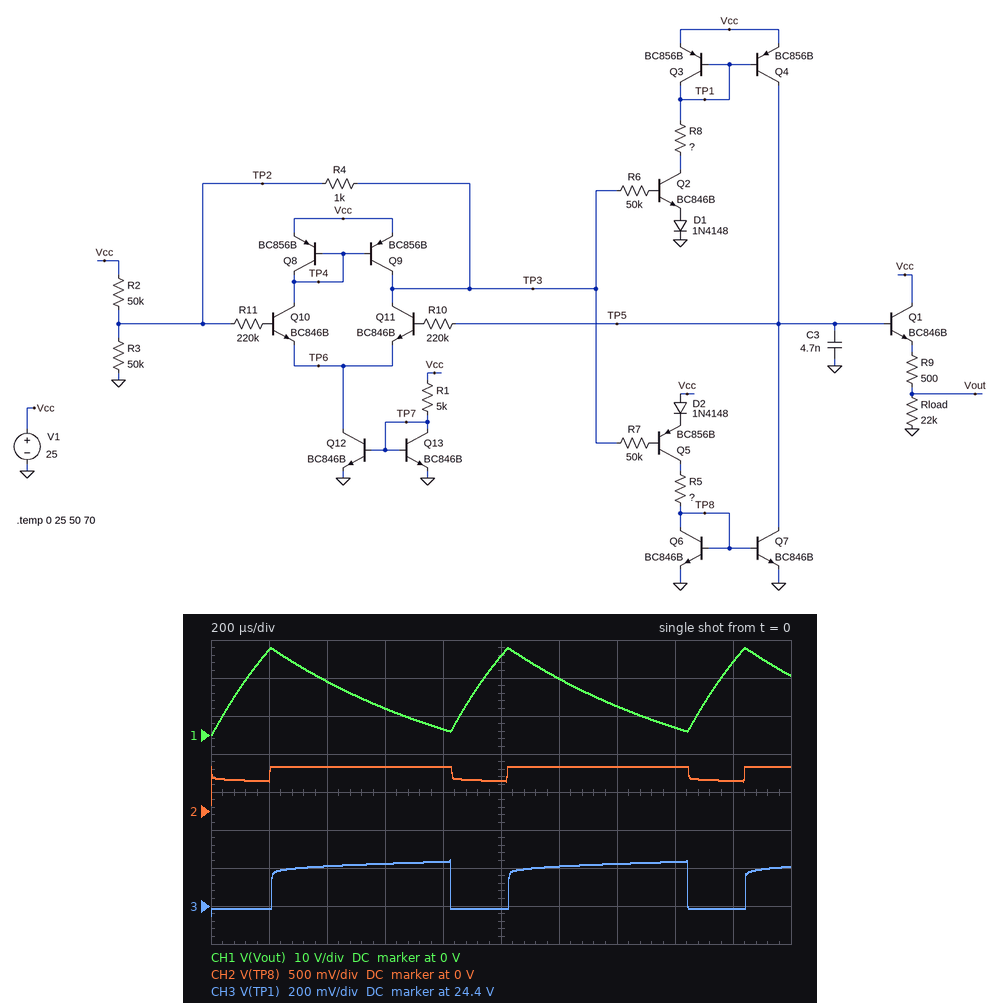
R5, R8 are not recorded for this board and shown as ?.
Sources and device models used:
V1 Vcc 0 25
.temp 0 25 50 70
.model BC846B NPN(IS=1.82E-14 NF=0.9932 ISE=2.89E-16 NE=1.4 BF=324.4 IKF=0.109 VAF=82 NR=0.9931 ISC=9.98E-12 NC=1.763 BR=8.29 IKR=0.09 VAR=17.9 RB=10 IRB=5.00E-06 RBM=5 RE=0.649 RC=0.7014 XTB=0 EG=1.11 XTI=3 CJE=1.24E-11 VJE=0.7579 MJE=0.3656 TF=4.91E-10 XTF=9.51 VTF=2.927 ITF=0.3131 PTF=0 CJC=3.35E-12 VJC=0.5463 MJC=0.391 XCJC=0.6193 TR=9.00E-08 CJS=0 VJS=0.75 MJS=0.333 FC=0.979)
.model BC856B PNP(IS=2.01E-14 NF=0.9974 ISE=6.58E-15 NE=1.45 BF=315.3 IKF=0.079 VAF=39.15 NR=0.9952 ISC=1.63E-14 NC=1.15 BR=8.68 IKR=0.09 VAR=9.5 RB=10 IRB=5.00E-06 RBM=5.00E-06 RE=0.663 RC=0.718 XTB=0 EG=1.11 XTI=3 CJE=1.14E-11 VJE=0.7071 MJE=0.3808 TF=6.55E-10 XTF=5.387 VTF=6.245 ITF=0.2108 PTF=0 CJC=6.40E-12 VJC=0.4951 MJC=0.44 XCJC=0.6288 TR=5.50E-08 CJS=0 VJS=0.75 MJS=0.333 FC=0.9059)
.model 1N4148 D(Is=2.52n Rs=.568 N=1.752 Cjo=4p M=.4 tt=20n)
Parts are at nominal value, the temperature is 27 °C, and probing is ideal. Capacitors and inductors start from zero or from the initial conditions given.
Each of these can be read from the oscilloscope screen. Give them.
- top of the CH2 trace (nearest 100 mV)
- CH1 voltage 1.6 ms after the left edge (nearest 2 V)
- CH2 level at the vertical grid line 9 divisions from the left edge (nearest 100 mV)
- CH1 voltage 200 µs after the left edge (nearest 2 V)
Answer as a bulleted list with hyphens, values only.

- 600 mV
- 2 V
- 400 mV
- 22 V
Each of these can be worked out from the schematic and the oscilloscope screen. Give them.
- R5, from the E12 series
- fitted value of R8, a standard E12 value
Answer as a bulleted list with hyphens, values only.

- 220 kΩ
- 56 kΩ
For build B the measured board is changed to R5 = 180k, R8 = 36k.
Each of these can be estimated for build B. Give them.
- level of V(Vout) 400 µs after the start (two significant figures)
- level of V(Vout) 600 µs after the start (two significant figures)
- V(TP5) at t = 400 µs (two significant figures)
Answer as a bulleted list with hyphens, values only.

- 10 V
- 3.0 V
- 11 V
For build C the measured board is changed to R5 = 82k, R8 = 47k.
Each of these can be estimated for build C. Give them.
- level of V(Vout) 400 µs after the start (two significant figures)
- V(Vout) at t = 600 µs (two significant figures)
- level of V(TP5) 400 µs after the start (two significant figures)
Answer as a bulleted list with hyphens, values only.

- 4.3 V
- 20 V
- 5.0 V
